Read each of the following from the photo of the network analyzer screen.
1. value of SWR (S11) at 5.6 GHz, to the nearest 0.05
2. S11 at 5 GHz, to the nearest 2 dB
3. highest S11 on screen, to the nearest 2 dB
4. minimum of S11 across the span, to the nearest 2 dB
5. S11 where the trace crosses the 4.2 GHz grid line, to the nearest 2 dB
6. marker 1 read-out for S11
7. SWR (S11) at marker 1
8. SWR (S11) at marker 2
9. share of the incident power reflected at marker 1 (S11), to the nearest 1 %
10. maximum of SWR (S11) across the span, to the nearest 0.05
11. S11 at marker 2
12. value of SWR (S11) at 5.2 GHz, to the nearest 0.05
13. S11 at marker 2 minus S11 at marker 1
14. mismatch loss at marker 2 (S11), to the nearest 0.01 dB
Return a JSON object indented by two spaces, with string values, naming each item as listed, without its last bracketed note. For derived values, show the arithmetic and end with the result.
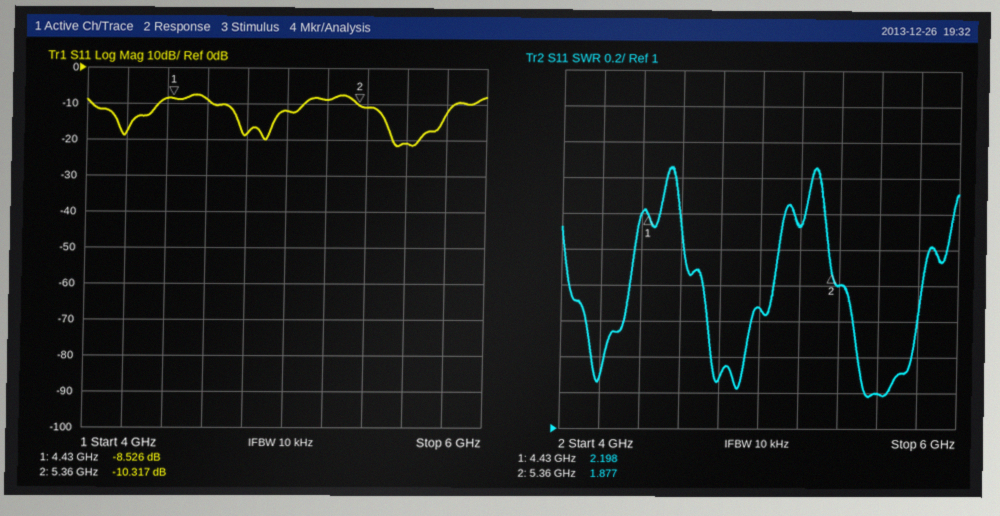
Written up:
{
  "value of SWR (S11) at 5.6 GHz, to the nearest 0.05": "1.20",
  "S11 at 5 GHz, to the nearest 2 dB": "-12 dB",
  "highest S11 on screen, to the nearest 2 dB": "-8 dB",
  "minimum of S11 across the span, to the nearest 2 dB": "-22 dB",
  "S11 where the trace crosses the 4.2 GHz grid line, to the nearest 2 dB": "-18 dB",
  "marker 1 read-out for S11": "-8.526 dB",
  "SWR (S11) at marker 1": "2.198",
  "SWR (S11) at marker 2": "1.877",
  "share of the incident power reflected at marker 1 (S11), to the nearest 1 %": "10^(-8.526/10) ≈ 14 %",
  "maximum of SWR (S11) across the span, to the nearest 0.05": "2.45",
  "S11 at marker 2": "-10.317 dB",
  "value of SWR (S11) at 5.2 GHz, to the nearest 0.05": "2.15",
  "S11 at marker 2 minus S11 at marker 1": "-10.317 − (-8.526) = -1.791 dB",
  "mismatch loss at marker 2 (S11), to the nearest 0.01 dB": "−10 log10(1 − 10^(-10.317/10)) ≈ 0.42 dB"
}
